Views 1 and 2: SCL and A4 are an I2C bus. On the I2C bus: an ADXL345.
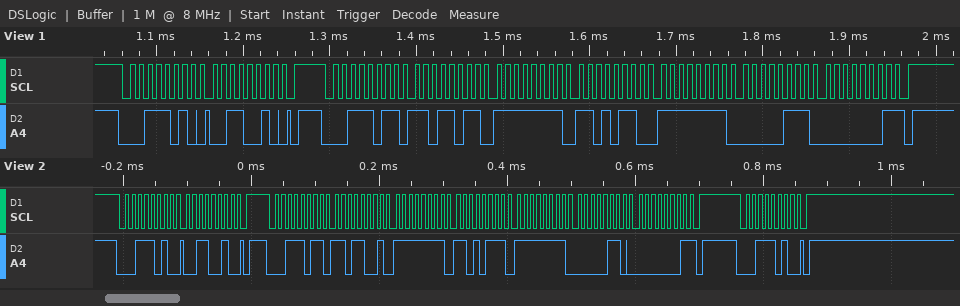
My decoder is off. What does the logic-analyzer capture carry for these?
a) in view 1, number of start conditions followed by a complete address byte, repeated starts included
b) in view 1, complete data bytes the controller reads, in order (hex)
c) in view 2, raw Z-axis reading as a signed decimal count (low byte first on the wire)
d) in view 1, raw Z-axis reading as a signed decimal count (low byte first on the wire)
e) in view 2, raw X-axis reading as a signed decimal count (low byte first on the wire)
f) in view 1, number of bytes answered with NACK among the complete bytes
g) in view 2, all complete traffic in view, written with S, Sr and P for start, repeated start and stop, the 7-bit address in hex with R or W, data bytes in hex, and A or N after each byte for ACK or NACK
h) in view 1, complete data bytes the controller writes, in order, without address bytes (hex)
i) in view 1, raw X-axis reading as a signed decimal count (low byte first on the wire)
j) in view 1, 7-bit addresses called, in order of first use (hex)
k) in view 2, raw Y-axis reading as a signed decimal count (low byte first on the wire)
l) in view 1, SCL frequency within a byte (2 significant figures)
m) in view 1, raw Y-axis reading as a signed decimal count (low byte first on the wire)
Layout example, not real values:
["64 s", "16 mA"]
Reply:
["2", "DB FF D6 FF 07 01", "262", "263", "-39", "1", "S 1DW A 32 A P S 1DR A D9 A FF A D7 A FF A 06 A 01 N P S 1DW A P", "32", "-37", "0x1D", "-41", "100 kHz", "-42"]
